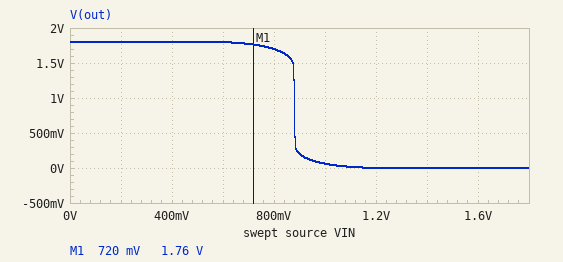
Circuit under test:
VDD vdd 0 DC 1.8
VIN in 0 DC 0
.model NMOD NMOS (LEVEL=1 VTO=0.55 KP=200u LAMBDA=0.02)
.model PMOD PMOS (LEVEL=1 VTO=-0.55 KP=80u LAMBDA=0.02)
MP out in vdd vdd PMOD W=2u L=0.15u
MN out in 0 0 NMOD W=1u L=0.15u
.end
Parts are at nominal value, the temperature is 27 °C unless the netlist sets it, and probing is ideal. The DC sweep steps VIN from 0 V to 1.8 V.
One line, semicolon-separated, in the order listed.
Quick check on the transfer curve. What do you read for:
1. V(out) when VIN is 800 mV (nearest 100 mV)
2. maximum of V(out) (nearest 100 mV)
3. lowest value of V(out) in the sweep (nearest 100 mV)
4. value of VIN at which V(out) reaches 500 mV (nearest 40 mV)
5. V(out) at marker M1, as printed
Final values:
1.7 V; 1.8 V; 0 V; 880 mV; 1.76 V
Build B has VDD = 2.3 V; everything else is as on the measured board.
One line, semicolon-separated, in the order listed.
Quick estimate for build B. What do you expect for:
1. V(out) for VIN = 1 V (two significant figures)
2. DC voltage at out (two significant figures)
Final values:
2.1 V; 2.3 V
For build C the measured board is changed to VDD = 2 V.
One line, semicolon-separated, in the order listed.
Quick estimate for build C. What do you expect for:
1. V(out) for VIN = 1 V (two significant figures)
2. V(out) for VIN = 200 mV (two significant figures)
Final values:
260 mV; 2.0 V
